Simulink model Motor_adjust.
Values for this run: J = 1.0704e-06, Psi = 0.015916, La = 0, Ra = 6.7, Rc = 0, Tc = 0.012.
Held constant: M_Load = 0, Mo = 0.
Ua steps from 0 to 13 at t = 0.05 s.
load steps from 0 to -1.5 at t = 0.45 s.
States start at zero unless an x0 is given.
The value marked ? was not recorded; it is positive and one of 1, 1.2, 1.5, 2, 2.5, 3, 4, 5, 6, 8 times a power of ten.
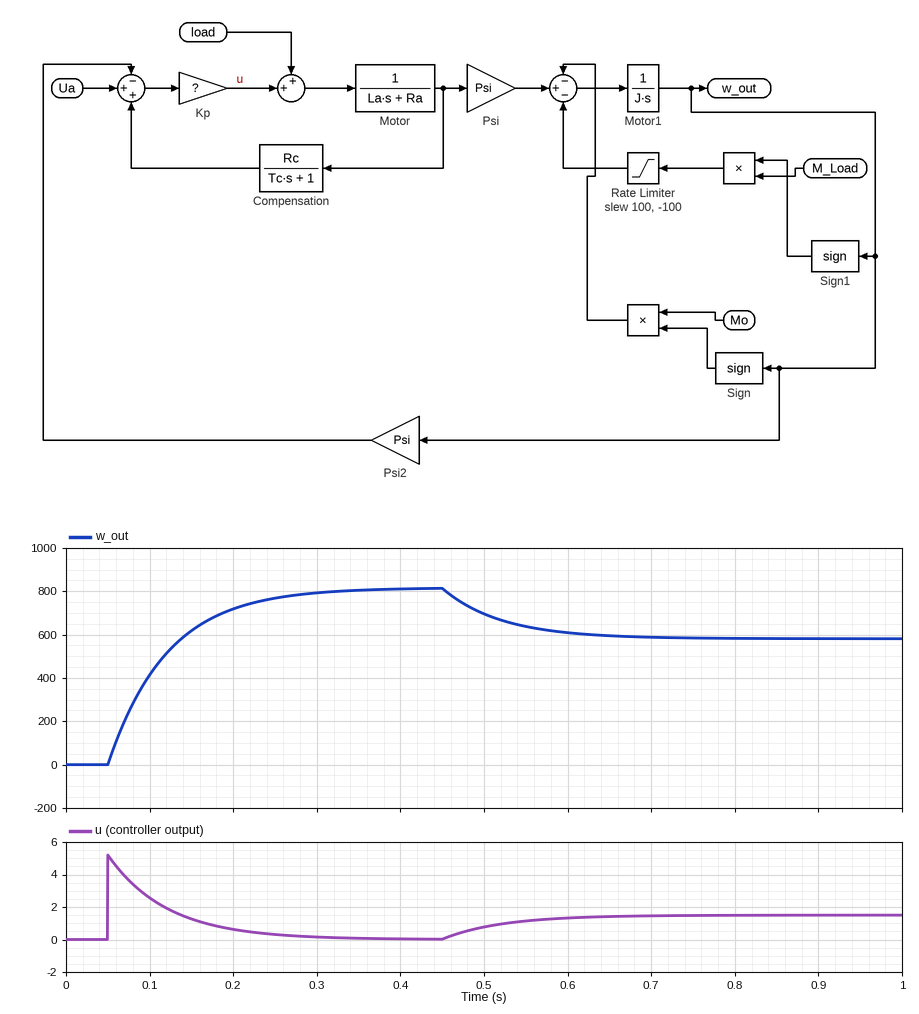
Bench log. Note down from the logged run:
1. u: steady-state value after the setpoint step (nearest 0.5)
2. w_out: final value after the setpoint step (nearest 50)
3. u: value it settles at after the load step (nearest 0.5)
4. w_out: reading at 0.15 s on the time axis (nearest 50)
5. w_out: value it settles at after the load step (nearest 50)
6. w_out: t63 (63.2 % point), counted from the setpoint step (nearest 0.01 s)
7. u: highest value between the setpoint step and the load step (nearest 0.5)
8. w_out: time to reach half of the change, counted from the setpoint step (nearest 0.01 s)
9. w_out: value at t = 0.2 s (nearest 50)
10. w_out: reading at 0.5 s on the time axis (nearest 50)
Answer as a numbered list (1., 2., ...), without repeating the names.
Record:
1. 0.0
2. 800
3. 1.5
4. 600
5. 600
6. 0.07 s
7. 5.0
8. 0.05 s
9. 700
10. 700
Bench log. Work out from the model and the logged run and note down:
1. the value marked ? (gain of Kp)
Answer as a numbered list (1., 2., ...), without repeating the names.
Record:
1. 0.4
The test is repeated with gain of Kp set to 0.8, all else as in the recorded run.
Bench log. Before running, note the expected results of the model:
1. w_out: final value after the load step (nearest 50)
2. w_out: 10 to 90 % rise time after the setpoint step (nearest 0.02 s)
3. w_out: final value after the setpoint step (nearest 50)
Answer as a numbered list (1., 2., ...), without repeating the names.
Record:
1. 700
2. 0.08 s
3. 800
